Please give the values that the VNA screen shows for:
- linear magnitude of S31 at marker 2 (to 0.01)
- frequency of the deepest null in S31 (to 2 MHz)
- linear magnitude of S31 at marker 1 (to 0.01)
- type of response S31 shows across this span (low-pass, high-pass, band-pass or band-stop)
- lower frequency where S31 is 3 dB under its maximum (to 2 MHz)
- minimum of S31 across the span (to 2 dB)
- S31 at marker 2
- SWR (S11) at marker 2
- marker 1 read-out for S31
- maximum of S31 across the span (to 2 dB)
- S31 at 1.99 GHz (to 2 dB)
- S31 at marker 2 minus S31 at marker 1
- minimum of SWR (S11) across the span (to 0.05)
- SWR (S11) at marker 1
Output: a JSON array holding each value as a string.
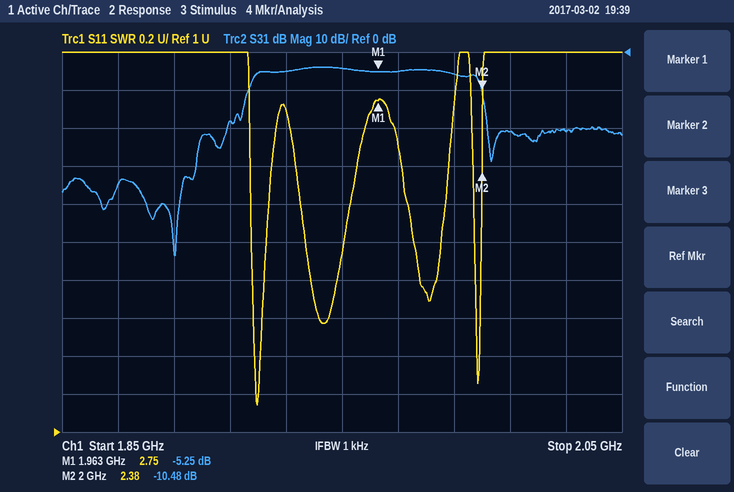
["0.30", "1.890 GHz", "0.55", "band-pass", "1.918 GHz", "-54 dB", "-10.48 dB", "2.38", "-5.25 dB", "-4 dB", "-6 dB", "-5.23 dB", "1.15", "2.75"]
